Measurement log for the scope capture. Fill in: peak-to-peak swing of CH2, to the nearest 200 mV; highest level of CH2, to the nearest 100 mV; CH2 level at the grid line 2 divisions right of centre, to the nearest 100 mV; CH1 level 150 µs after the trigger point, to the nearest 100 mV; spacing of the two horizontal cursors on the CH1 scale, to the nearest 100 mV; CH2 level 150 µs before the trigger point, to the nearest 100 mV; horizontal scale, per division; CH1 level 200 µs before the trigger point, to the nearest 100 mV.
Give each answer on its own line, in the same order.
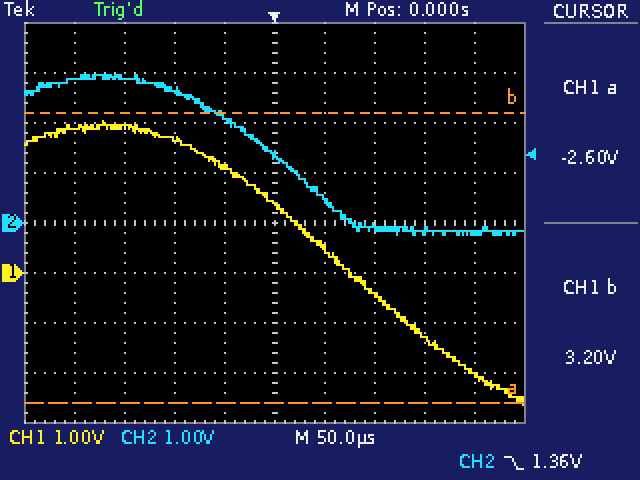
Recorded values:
3.2 V
3.0 V
-100 mV
-1.3 V
5.8 V
2.9 V
50 µs
2.9 V
